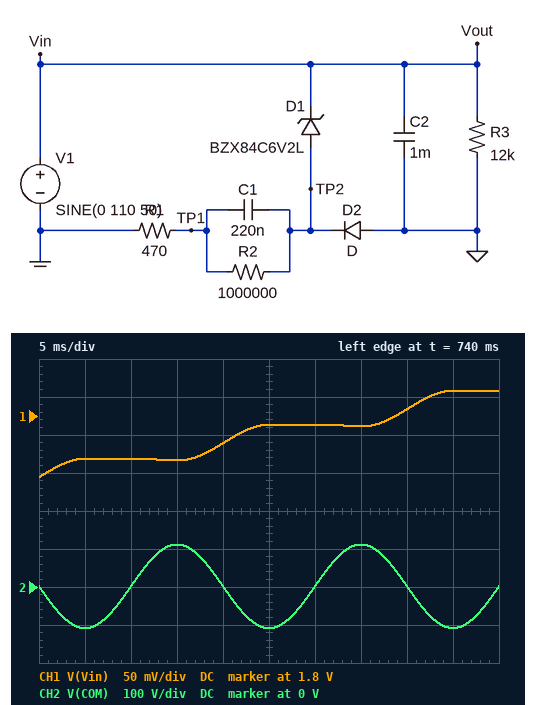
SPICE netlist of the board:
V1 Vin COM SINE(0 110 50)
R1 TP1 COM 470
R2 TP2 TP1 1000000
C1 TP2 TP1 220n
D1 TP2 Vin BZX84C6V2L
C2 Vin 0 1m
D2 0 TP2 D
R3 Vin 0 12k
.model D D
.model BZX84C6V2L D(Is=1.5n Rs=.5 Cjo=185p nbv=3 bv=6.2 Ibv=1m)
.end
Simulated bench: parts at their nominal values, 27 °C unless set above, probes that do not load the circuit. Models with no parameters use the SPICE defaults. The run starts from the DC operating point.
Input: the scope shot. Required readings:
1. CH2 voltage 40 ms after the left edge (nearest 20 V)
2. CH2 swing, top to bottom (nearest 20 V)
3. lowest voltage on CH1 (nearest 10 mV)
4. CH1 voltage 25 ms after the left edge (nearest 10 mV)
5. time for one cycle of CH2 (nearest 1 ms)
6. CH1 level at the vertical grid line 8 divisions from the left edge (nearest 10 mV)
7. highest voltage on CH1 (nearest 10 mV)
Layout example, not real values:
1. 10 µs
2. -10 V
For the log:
1. 0 V
2. 220 V
3. 1.72 V
4. 1.79 V
5. 20 ms
6. 1.81 V
7. 1.83 V
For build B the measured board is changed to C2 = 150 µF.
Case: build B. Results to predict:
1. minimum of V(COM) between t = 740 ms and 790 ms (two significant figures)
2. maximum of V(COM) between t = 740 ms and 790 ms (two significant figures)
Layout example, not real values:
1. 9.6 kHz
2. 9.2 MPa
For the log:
1. -100 V
2. 120 V
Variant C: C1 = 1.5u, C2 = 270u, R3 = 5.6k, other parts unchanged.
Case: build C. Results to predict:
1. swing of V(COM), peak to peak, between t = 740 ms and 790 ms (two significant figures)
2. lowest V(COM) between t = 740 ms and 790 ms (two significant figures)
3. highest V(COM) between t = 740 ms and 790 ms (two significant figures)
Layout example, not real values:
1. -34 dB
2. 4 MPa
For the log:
1. 220 V
2. -100 V
3. 120 V
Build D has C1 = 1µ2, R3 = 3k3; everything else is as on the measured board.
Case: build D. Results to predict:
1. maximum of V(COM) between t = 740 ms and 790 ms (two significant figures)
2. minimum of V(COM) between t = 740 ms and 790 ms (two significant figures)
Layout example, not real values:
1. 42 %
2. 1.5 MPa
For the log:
1. 120 V
2. -100 V
